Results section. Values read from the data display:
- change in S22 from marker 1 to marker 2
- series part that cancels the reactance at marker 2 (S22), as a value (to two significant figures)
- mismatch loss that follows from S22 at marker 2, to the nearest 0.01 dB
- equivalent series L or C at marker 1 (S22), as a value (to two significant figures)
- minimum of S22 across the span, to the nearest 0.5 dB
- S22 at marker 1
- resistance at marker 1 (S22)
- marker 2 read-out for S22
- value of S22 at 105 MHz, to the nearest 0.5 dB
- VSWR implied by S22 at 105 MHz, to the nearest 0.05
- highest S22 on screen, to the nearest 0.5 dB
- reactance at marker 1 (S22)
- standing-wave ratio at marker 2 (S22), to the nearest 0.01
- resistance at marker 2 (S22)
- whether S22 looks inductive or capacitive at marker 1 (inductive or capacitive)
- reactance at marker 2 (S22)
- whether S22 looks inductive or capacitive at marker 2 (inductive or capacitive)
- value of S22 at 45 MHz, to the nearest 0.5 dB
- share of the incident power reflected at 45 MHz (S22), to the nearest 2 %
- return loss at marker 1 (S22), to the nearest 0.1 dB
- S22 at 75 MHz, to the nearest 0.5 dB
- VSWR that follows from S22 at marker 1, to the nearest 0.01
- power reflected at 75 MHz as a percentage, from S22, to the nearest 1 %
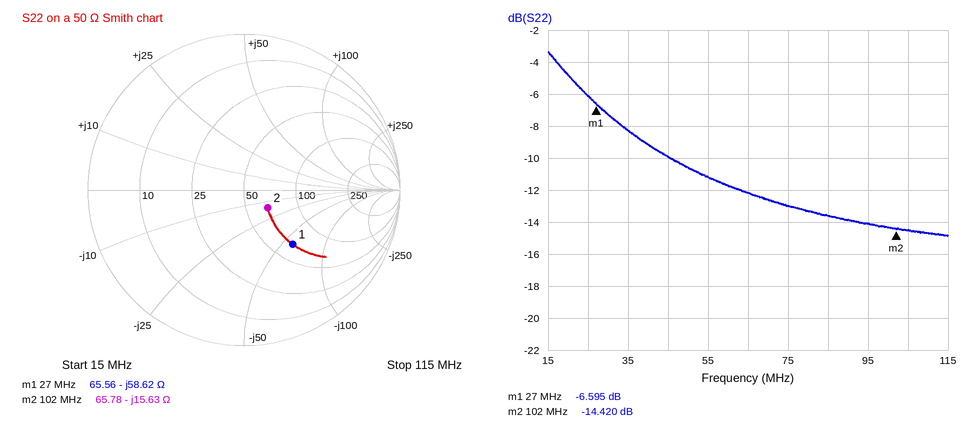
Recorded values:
-7.825 dB
24 nH
0.16 dB
100 pF
-15.0 dB
-6.595 dB
65.56 Ω
-14.420 dB
-14.5 dB
1.45
-3.5 dB
-58.62 Ω
1.47
65.78 Ω
capacitive
-15.63 Ω
capacitive
-10.0 dB
10 %
6.6 dB
-13.0 dB
2.76
5 %
